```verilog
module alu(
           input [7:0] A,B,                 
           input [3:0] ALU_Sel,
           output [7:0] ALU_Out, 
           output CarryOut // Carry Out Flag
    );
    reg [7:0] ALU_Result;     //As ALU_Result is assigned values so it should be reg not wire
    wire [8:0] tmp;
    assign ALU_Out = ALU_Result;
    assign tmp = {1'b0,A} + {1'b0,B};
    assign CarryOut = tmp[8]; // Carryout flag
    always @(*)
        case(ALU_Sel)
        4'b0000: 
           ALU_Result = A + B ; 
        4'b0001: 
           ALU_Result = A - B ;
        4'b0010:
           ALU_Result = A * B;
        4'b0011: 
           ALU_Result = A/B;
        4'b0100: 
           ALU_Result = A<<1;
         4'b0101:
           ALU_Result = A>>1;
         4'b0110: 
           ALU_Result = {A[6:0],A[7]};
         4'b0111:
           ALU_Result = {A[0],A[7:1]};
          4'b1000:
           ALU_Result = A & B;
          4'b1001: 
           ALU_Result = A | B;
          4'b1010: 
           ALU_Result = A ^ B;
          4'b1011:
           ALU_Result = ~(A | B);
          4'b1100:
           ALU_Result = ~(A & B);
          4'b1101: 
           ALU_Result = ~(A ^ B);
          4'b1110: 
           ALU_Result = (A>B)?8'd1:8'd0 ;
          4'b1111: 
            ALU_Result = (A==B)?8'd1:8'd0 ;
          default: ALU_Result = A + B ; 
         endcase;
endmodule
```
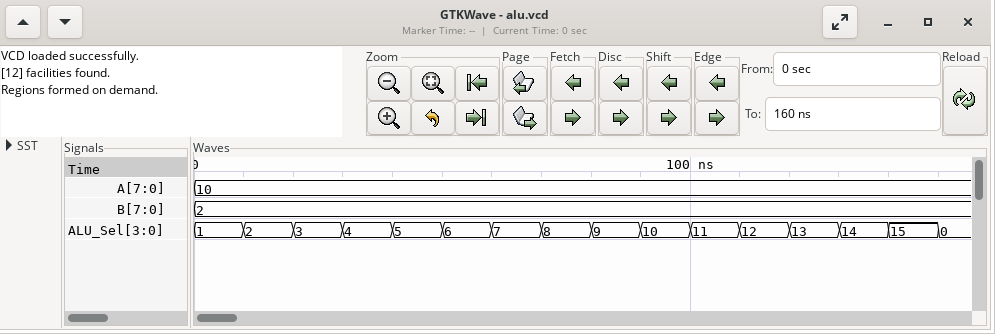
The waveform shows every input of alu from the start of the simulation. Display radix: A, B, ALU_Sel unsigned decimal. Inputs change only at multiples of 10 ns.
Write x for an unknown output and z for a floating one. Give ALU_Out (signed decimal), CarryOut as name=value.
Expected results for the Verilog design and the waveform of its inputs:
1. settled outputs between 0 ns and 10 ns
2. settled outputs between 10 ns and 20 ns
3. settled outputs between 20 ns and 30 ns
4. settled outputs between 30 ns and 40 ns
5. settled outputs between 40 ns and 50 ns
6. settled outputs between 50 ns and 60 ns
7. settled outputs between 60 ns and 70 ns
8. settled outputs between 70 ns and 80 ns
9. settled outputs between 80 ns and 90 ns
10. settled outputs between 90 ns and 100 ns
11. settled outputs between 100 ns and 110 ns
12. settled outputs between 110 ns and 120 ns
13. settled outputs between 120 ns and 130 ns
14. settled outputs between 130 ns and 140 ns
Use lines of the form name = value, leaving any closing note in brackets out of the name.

settled outputs between 0 ns and 10 ns = ALU_Out=8, CarryOut=0
settled outputs between 10 ns and 20 ns = ALU_Out=20, CarryOut=0
settled outputs between 20 ns and 30 ns = ALU_Out=5, CarryOut=0
settled outputs between 30 ns and 40 ns = ALU_Out=20, CarryOut=0
settled outputs between 40 ns and 50 ns = ALU_Out=5, CarryOut=0
settled outputs between 50 ns and 60 ns = ALU_Out=20, CarryOut=0
settled outputs between 60 ns and 70 ns = ALU_Out=5, CarryOut=0
settled outputs between 70 ns and 80 ns = ALU_Out=2, CarryOut=0
settled outputs between 80 ns and 90 ns = ALU_Out=10, CarryOut=0
settled outputs between 90 ns and 100 ns = ALU_Out=8, CarryOut=0
settled outputs between 100 ns and 110 ns = ALU_Out=-11, CarryOut=0
settled outputs between 110 ns and 120 ns = ALU_Out=-3, CarryOut=0
settled outputs between 120 ns and 130 ns = ALU_Out=-9, CarryOut=0
settled outputs between 130 ns and 140 ns = ALU_Out=1, CarryOut=0
